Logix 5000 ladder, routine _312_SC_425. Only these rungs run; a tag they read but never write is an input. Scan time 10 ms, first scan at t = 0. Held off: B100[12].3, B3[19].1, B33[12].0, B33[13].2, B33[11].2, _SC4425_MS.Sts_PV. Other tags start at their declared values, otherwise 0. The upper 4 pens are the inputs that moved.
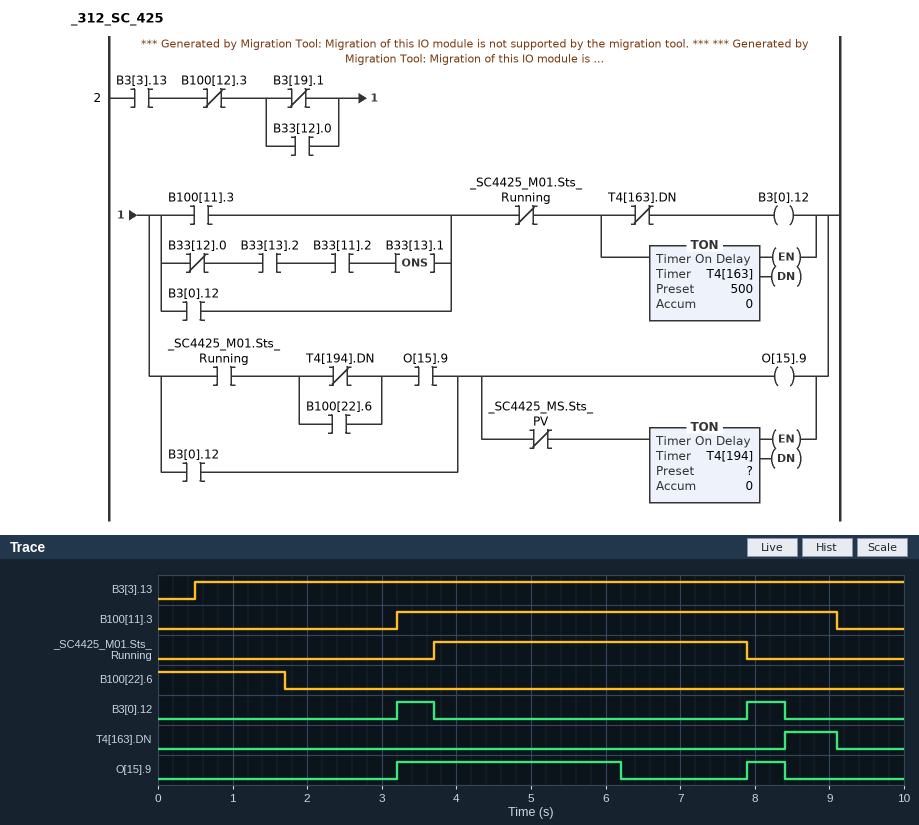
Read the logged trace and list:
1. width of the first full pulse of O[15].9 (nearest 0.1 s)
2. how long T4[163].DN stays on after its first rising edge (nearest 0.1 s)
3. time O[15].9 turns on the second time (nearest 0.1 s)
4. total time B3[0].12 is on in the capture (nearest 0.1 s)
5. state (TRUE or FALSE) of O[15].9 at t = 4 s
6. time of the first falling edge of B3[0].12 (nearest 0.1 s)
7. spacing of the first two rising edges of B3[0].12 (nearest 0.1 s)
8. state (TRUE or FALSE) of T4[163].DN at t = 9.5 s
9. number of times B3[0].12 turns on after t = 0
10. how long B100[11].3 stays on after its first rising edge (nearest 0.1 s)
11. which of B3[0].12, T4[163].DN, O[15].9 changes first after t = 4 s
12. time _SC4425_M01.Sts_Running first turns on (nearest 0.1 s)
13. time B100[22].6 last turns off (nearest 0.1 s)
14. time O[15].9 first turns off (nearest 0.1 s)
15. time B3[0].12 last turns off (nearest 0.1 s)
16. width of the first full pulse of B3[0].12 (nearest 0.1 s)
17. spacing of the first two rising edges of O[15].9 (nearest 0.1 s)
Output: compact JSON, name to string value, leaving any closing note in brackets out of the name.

{"width of the first full pulse of O[15].9": "3.0 s", "how long T4[163].DN stays on after its first rising edge": "0.7 s", "time O[15].9 turns on the second time": "7.9 s", "total time B3[0].12 is on in the capture": "1.0 s", "state (TRUE or FALSE) of O[15].9 at t = 4 s": "TRUE", "time of the first falling edge of B3[0].12": "3.7 s", "spacing of the first two rising edges of B3[0].12": "4.7 s", "state (TRUE or FALSE) of T4[163].DN at t = 9.5 s": "FALSE", "number of times B3[0].12 turns on after t = 0": "2", "how long B100[11].3 stays on after its first rising edge": "5.9 s", "which of B3[0].12, T4[163].DN, O[15].9 changes first after t = 4 s": "O[15].9", "time _SC4425_M01.Sts_Running first turns on": "3.7 s", "time B100[22].6 last turns off": "1.7 s", "time O[15].9 first turns off": "6.2 s", "time B3[0].12 last turns off": "8.4 s", "width of the first full pulse of B3[0].12": "0.5 s", "spacing of the first two rising edges of O[15].9": "4.7 s"}
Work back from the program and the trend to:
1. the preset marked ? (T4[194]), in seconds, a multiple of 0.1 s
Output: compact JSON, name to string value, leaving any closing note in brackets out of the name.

{"the preset marked ? (T4[194]), in seconds, a multiple of 0.1 s": "3.0 s"}
